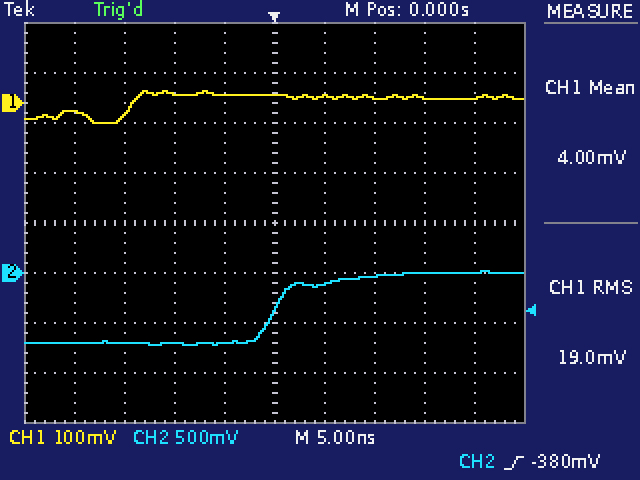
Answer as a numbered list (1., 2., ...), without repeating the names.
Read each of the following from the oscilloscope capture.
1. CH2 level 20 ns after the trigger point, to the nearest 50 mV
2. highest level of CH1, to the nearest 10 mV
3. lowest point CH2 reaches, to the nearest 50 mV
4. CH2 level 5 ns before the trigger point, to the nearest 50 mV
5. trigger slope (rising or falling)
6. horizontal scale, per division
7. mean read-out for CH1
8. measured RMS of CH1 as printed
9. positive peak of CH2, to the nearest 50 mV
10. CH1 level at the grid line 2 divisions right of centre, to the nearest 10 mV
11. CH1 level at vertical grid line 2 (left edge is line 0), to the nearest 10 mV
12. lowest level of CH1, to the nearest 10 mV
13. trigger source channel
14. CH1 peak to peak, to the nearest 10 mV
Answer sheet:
1. 0 mV
2. 20 mV
3. -700 mV
4. -700 mV
5. rising
6. 5 ns
7. 4.00 mV
8. 19.0 mV
9. 0 mV
10. 10 mV
11. -20 mV
12. -40 mV
13. CH2
14. 60 mV
